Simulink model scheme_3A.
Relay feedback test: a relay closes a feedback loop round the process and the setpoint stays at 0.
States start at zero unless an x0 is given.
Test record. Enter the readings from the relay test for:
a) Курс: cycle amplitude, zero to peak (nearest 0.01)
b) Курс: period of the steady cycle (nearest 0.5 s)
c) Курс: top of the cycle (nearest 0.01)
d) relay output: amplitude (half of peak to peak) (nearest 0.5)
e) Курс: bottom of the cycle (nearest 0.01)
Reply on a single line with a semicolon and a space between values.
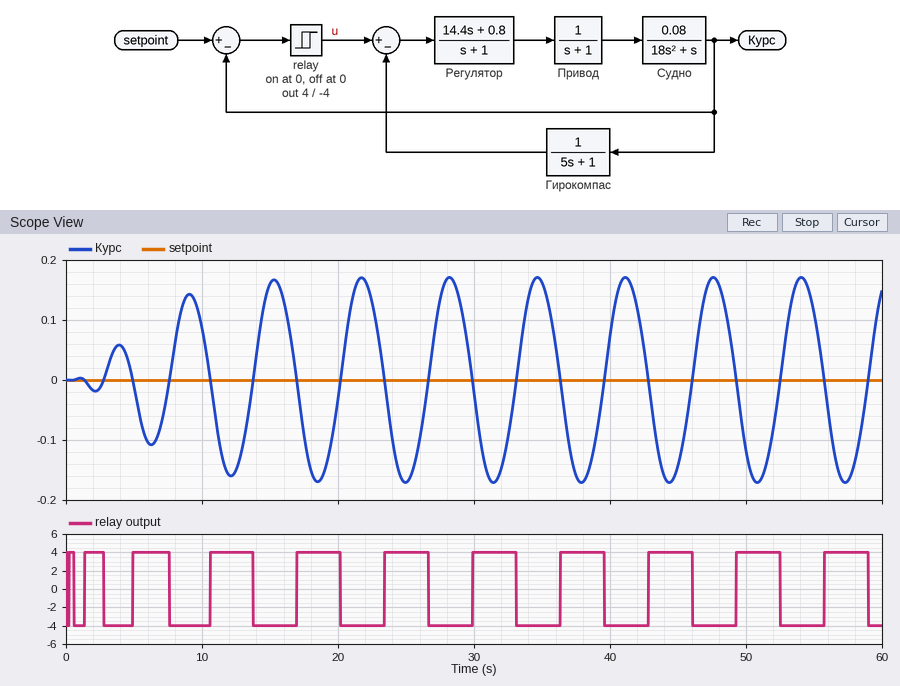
0.17; 6.5 s; 0.17; 4.0; -0.17
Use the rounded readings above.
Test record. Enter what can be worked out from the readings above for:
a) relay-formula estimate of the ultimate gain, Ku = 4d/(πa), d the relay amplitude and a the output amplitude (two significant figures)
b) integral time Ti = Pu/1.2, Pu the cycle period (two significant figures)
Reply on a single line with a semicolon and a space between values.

30; 5.4 s
